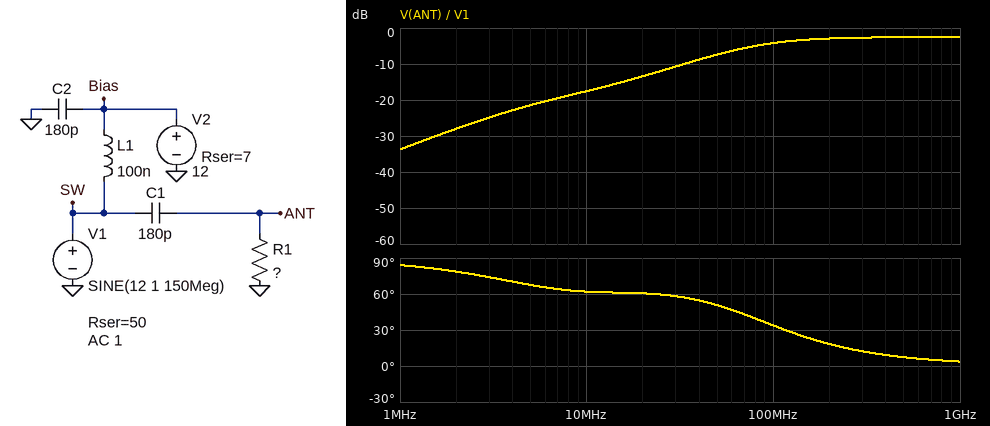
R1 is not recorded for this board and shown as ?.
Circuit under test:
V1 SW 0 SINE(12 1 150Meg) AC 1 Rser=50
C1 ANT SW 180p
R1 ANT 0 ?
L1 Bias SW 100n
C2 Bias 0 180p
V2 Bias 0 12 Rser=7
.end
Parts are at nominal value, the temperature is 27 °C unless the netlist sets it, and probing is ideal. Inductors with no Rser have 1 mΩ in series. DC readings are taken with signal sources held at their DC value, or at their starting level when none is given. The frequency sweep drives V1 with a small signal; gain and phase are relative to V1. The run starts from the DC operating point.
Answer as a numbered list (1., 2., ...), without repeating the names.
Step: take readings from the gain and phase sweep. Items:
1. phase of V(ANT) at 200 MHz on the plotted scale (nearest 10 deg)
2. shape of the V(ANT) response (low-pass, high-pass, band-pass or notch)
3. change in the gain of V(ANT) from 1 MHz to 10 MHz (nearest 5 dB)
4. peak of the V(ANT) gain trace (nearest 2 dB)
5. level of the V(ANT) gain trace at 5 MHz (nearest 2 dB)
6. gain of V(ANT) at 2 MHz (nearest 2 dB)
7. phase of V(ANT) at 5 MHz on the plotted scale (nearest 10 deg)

1. 20 deg
2. high-pass
3. 15 dB
4. -2 dB
5. -22 dB
6. -28 dB
7. 70 deg
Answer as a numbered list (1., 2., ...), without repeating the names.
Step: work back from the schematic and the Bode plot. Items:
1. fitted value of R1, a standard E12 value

1. 150 Ω
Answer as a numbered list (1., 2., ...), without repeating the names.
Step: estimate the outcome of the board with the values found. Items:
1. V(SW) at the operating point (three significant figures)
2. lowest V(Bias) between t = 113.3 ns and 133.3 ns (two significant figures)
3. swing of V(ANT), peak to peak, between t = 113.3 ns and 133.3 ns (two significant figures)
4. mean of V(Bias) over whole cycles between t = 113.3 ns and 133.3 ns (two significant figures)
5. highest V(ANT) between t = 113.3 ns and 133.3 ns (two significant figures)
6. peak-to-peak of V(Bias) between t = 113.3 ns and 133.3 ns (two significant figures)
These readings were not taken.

1. 12.0 V
2. 12 V
3. 1.4 V
4. 12 V
5. 690 mV
6. 68 mV
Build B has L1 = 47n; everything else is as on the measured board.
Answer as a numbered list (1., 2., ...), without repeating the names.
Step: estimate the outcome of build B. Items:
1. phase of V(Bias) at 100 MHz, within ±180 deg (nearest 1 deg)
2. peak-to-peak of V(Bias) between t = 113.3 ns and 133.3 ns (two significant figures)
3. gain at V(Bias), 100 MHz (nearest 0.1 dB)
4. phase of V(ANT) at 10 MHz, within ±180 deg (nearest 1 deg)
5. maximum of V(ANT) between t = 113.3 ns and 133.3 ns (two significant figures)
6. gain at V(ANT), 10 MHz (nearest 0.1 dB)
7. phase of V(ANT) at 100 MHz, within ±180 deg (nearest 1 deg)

1. -71 deg
2. 120 mV
3. -21.5 dB
4. 46 deg
5. 540 mV
6. -19.3 dB
7. 52 deg
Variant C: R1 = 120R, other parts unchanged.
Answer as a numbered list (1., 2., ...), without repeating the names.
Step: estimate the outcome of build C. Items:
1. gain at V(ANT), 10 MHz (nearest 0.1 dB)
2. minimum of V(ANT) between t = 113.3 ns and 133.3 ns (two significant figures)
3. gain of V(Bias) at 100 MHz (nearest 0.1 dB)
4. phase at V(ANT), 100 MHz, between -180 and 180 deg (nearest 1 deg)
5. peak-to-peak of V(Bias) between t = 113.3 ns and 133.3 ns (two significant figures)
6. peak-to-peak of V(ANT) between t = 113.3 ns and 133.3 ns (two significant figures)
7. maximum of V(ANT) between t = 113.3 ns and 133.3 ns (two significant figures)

1. -18.1 dB
2. -650 mV
3. -25.2 dB
4. 33 deg
5. 65 mV
6. 1.3 V
7. 650 mV
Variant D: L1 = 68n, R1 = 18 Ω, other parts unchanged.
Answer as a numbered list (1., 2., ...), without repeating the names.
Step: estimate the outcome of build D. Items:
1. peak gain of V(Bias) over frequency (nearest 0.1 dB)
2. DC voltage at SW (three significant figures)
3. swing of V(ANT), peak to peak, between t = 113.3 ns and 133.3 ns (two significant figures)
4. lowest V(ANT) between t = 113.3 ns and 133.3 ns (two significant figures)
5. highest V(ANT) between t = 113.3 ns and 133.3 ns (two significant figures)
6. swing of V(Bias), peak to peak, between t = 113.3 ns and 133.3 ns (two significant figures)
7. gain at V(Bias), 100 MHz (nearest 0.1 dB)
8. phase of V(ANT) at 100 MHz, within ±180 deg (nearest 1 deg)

1. -18.0 dB
2. 12.0 V
3. 540 mV
4. -270 mV
5. 270 mV
6. 42 mV
7. -27.7 dB
8. 29 deg
